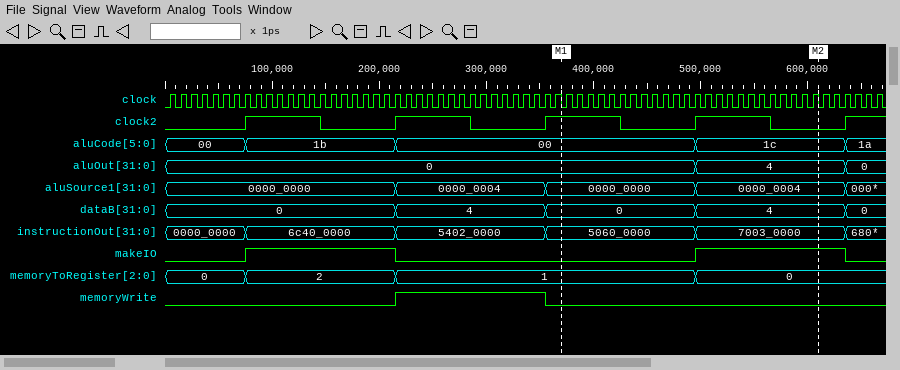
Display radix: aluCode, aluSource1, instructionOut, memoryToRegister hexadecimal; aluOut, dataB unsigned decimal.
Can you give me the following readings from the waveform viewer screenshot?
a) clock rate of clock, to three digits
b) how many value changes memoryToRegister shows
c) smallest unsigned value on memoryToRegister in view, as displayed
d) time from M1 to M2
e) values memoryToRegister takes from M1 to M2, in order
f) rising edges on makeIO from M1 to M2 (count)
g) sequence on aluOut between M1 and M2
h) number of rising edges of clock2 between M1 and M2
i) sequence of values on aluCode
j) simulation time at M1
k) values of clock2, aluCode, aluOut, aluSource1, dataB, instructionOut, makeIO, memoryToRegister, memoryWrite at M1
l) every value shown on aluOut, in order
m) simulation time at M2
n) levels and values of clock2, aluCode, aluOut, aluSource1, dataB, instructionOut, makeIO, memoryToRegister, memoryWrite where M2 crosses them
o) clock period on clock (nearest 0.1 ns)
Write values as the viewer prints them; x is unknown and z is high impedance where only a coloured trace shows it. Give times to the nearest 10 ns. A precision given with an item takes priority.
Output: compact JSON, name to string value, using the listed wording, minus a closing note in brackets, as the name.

{"clock rate of clock, to three digits": "100 MHz", "how many value changes memoryToRegister shows": "3", "smallest unsigned value on memoryToRegister in view, as displayed": "0", "time from M1 to M2": "240 ns", "values memoryToRegister takes from M1 to M2, in order": "1, 0", "rising edges on makeIO from M1 to M2": "1", "sequence on aluOut between M1 and M2": "0, 4", "number of rising edges of clock2 between M1 and M2": "1", "sequence of values on aluCode": "00, 1b, 00, 1c, 1a", "simulation time at M1": "370 ns", "values of clock2, aluCode, aluOut, aluSource1, dataB, instructionOut, makeIO, memoryToRegister, memoryWrite at M1": "clock2=1, aluCode=00, aluOut=0, aluSource1=0000_0000, dataB=0, instructionOut=5060_0000, makeIO=0, memoryToRegister=1, memoryWrite=0", "every value shown on aluOut, in order": "0, 4, 0", "simulation time at M2": "610 ns", "levels and values of clock2, aluCode, aluOut, aluSource1, dataB, instructionOut, makeIO, memoryToRegister, memoryWrite where M2 crosses them": "clock2=0, aluCode=1c, aluOut=4, aluSource1=0000_0004, dataB=4, instructionOut=7003_0000, makeIO=1, memoryToRegister=0, memoryWrite=0", "clock period on clock": "10 ns"}
